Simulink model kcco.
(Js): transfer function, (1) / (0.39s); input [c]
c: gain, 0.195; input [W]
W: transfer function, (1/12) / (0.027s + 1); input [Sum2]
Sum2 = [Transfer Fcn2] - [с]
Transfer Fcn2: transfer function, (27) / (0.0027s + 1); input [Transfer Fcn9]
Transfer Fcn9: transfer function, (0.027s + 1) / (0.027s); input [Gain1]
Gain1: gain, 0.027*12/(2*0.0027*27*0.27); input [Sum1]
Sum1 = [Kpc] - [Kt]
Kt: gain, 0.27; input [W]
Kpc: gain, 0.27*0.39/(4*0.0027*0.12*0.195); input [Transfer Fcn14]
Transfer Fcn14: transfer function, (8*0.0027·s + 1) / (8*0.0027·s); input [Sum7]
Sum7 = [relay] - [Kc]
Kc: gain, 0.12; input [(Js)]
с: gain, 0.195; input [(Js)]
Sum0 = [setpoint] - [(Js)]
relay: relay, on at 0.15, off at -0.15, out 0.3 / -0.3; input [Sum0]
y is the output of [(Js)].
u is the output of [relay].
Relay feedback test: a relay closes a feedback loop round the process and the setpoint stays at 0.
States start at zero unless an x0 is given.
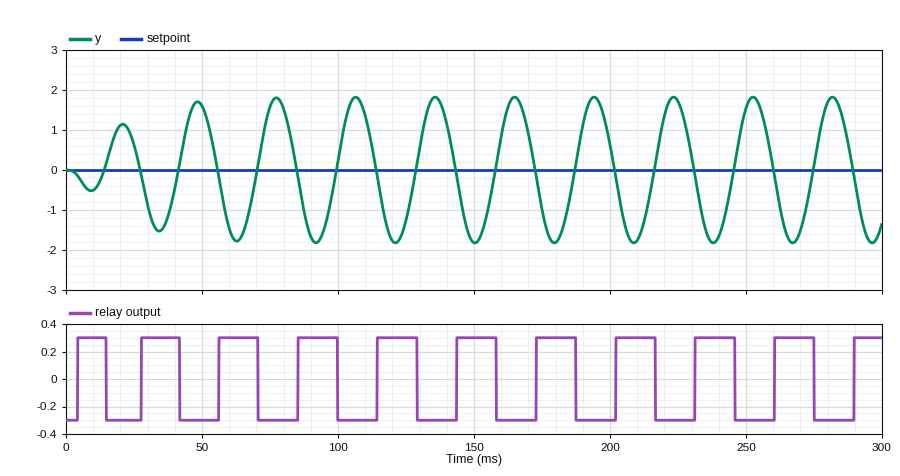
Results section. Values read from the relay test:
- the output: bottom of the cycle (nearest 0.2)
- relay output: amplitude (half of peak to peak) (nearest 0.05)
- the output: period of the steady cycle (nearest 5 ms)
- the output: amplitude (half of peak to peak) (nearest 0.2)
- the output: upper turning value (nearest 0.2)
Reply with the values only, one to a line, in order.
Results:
-1.8
0.30
30 ms
1.8
1.8
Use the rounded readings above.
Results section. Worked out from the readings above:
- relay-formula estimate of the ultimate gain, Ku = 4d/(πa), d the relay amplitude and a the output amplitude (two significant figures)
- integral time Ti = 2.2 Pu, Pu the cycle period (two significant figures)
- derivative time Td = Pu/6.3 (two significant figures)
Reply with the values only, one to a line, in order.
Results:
0.21
66 ms
4.8 ms
